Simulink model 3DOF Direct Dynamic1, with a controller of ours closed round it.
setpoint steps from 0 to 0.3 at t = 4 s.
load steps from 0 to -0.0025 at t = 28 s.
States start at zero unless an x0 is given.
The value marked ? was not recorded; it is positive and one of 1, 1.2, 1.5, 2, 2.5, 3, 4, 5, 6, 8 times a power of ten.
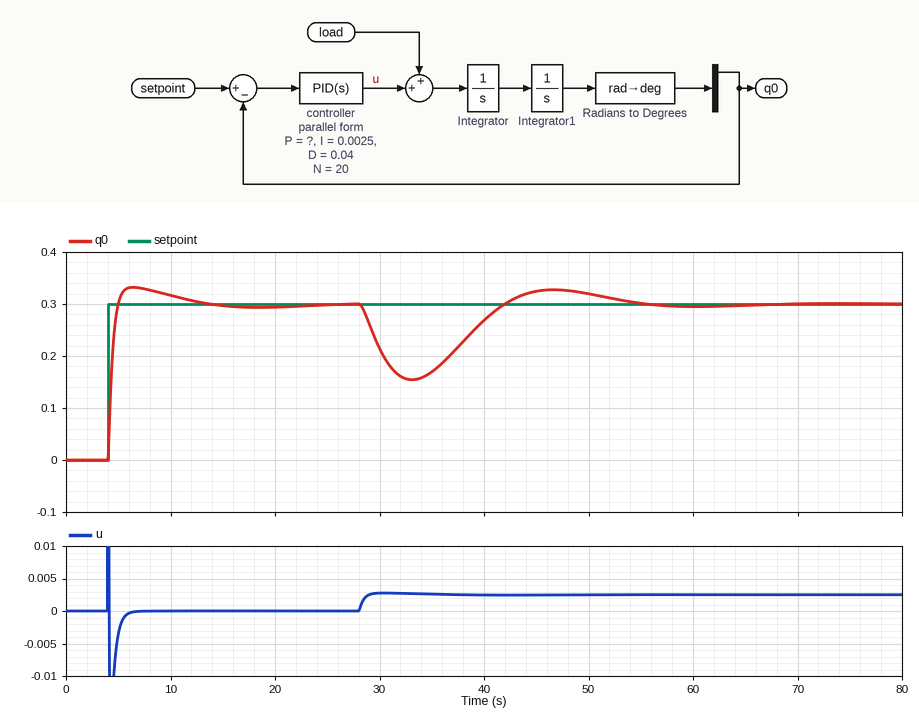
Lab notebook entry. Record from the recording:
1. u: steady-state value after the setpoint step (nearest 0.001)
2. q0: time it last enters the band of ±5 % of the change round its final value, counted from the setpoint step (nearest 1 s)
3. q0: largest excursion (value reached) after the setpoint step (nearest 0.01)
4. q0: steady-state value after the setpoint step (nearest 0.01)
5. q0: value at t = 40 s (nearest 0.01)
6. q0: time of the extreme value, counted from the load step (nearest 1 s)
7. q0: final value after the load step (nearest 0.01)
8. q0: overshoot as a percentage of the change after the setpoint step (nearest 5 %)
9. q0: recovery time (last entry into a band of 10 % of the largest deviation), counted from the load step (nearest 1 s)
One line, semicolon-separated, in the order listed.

0.000; 6 s; 0.33; 0.30; 0.27; 5 s; 0.30; 10 %; 23 s
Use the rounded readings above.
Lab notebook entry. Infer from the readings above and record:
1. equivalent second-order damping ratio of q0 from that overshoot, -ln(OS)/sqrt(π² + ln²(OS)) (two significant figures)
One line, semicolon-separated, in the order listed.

0.59
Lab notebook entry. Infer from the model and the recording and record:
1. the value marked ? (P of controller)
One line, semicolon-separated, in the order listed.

0.01
